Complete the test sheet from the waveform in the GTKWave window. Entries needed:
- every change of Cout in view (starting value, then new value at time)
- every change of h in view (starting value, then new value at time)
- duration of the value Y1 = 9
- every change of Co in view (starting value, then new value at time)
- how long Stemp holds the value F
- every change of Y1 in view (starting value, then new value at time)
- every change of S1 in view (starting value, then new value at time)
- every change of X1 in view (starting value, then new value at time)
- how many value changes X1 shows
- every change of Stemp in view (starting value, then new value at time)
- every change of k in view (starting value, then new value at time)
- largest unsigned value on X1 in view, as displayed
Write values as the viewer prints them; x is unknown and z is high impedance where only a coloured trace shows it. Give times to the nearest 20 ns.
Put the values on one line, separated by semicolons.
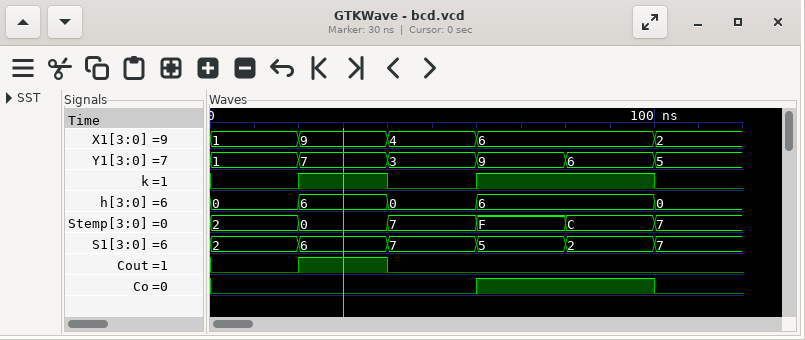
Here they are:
0, 1 at 20 ns, 0 at 40 ns; 0, 6 at 20 ns, 0 at 40 ns, 6 at 60 ns, 0 at 100 ns; 20 ns; 0, 1 at 60 ns, 0 at 100 ns; 20 ns; 1, 7 at 20 ns, 3 at 40 ns, 9 at 60 ns, 6 at 80 ns, 5 at 100 ns; 2, 6 at 20 ns, 7 at 40 ns, 5 at 60 ns, 2 at 80 ns, 7 at 100 ns; 1, 9 at 20 ns, 4 at 40 ns, 6 at 60 ns, 2 at 100 ns; 4; 2, 0 at 20 ns, 7 at 40 ns, F at 60 ns, C at 80 ns, 7 at 100 ns; 0, 1 at 20 ns, 0 at 40 ns, 1 at 60 ns, 0 at 100 ns; 9
